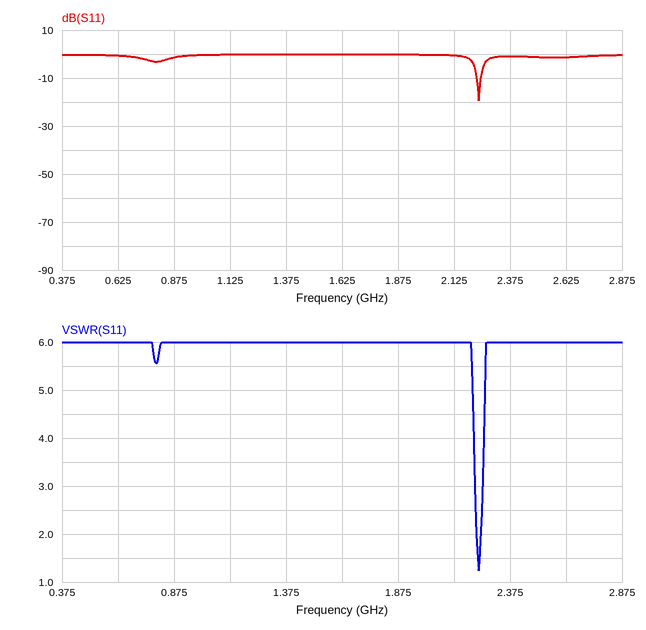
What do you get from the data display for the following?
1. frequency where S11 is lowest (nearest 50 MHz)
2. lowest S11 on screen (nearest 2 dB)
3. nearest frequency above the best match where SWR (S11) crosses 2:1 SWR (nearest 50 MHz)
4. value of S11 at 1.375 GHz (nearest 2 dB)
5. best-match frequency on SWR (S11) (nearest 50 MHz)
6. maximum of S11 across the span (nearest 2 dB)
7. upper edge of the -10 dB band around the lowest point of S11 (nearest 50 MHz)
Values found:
2.25 GHz
-20 dB
2.25 GHz
0 dB
2.25 GHz
0 dB
2.25 GHz
